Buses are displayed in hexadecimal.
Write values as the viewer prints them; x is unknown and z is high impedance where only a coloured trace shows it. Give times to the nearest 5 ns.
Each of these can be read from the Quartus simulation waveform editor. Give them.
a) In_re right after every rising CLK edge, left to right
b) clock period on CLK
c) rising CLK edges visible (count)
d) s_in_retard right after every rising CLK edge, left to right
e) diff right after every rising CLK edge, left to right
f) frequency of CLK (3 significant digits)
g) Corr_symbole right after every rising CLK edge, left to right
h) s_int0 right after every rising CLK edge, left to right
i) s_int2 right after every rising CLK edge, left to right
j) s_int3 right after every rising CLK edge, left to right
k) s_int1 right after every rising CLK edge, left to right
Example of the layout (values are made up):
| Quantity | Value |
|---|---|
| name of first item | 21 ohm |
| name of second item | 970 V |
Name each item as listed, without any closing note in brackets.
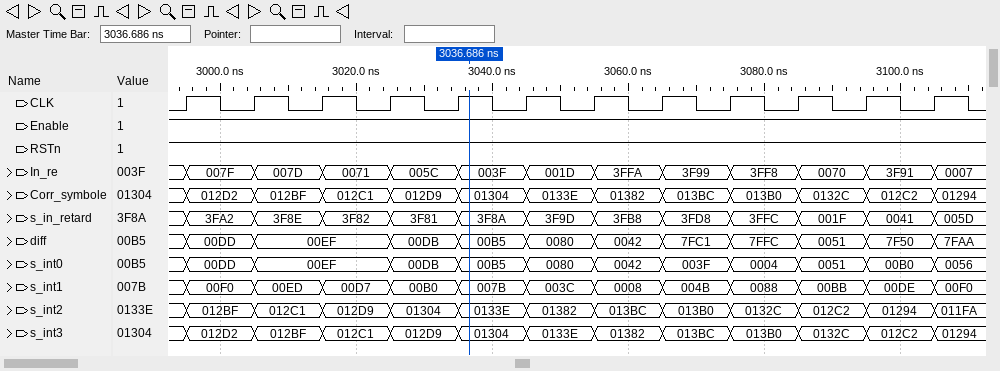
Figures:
| Quantity | Value |
|---|---|
| In_re right after every rising CLK edge, left to right | 007F, 007D, 0071, 005C, 003F, 001D, 3FFA, 3F99, 3FF8, 0070, 3F91, 0007 |
| clock period on CLK | 10 ns |
| rising CLK edges visible | 12 |
| s_in_retard right after every rising CLK edge, left to right | 3FA2, 3F8E, 3F82, 3F81, 3F8A, 3F9D, 3FB8, 3FD8, 3FFC, 001F, 0041, 005D |
| diff right after every rising CLK edge, left to right | 00DD, 00EF, 00EF, 00DB, 00B5, 0080, 0042, 7FC1, 7FFC, 0051, 7F50, 7FAA |
| frequency of CLK | 100 MHz |
| Corr_symbole right after every rising CLK edge, left to right | 012D2, 012BF, 012C1, 012D9, 01304, 0133E, 01382, 013BC, 013B0, 0132C, 012C2, 01294 |
| s_int0 right after every rising CLK edge, left to right | 00DD, 00EF, 00EF, 00DB, 00B5, 0080, 0042, 003F, 0004, 0051, 00B0, 0056 |
| s_int2 right after every rising CLK edge, left to right | 012BF, 012C1, 012D9, 01304, 0133E, 01382, 013BC, 013B0, 0132C, 012C2, 01294, 011FA |
| s_int3 right after every rising CLK edge, left to right | 012D2, 012BF, 012C1, 012D9, 01304, 0133E, 01382, 013BC, 013B0, 0132C, 012C2, 01294 |
| s_int1 right after every rising CLK edge, left to right | 00F0, 00ED, 00D7, 00B0, 007B, 003C, 0008, 004B, 0088, 00BB, 00DE, 00F0 |
